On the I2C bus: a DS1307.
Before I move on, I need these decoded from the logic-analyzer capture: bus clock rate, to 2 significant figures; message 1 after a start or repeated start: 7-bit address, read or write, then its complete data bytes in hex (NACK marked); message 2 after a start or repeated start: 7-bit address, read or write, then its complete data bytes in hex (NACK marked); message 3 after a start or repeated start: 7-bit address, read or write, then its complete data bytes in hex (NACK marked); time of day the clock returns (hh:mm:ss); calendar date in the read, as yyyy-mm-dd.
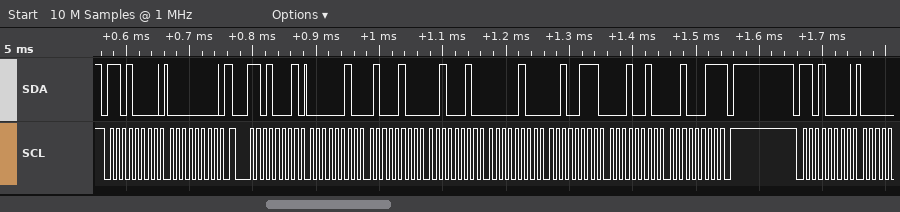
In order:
100 kHz
0x68 write: 00
0x68 read: 02 44 22 04 27 12 23 NACK
0x68 write
22:44:02
2023-12-27
